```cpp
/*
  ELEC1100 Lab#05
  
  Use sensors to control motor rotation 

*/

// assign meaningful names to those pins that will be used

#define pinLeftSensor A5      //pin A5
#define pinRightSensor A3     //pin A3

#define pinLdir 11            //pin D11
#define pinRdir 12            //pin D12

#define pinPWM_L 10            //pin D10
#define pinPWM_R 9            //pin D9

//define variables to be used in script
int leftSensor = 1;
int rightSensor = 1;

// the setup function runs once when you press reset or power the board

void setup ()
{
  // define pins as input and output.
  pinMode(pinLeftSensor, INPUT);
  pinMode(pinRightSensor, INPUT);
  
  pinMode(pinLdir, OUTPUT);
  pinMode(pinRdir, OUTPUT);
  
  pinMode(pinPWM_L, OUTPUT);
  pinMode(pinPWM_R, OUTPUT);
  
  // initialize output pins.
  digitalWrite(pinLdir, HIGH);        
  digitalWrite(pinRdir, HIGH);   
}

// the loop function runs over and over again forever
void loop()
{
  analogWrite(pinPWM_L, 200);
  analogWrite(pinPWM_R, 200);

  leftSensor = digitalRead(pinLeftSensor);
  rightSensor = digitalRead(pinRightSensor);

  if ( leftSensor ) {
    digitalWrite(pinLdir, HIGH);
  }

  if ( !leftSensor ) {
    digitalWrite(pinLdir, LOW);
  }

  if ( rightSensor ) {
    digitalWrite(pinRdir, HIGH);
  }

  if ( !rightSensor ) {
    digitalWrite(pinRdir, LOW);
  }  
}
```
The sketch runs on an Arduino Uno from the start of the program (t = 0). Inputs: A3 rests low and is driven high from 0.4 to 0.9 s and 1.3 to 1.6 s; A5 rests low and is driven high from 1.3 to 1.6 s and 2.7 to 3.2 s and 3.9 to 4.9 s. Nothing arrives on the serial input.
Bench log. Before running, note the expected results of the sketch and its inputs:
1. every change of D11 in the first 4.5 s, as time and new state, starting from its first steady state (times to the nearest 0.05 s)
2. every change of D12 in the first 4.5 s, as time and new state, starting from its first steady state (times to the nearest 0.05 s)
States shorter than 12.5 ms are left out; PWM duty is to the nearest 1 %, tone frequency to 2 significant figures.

0 s low; 1.3 s high; 1.6 s low; 2.7 s high; 3.2 s low; 3.9 s high
0 s low; 0.4 s high; 0.9 s low; 1.3 s high; 1.6 s low
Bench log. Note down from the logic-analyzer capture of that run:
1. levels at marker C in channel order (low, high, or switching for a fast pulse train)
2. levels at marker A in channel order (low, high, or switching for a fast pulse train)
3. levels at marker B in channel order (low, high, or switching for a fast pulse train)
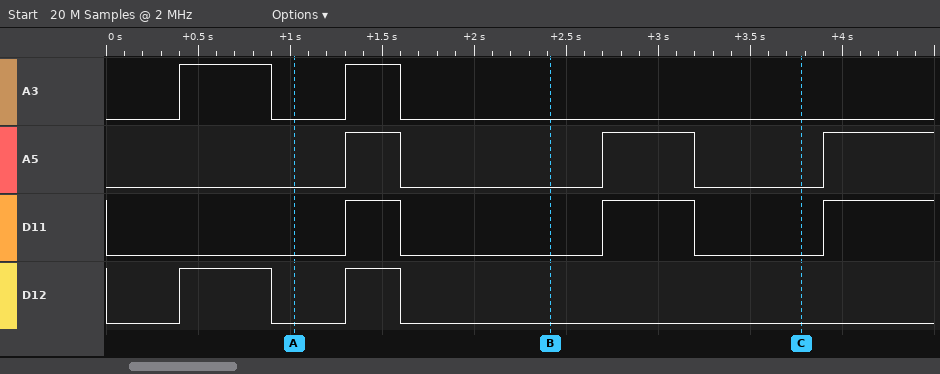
A3 low, A5 low, D11 low, D12 low
A3 low, A5 low, D11 low, D12 low
A3 low, A5 low, D11 low, D12 low
